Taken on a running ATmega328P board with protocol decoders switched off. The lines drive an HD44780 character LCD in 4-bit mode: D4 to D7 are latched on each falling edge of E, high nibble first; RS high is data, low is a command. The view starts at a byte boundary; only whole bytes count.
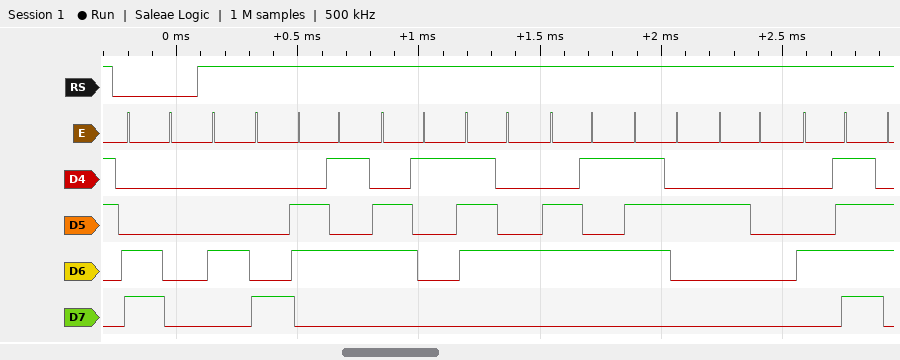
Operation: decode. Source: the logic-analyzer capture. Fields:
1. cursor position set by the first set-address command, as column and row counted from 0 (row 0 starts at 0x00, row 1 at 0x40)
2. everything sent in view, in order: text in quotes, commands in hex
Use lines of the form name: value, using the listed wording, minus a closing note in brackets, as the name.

cursor position set by the first set-address command, as column and row counted from 0: column 0, row 1
everything sent in view, in order: text in quotes, commands in hex: 0xC0 "Heater O"
